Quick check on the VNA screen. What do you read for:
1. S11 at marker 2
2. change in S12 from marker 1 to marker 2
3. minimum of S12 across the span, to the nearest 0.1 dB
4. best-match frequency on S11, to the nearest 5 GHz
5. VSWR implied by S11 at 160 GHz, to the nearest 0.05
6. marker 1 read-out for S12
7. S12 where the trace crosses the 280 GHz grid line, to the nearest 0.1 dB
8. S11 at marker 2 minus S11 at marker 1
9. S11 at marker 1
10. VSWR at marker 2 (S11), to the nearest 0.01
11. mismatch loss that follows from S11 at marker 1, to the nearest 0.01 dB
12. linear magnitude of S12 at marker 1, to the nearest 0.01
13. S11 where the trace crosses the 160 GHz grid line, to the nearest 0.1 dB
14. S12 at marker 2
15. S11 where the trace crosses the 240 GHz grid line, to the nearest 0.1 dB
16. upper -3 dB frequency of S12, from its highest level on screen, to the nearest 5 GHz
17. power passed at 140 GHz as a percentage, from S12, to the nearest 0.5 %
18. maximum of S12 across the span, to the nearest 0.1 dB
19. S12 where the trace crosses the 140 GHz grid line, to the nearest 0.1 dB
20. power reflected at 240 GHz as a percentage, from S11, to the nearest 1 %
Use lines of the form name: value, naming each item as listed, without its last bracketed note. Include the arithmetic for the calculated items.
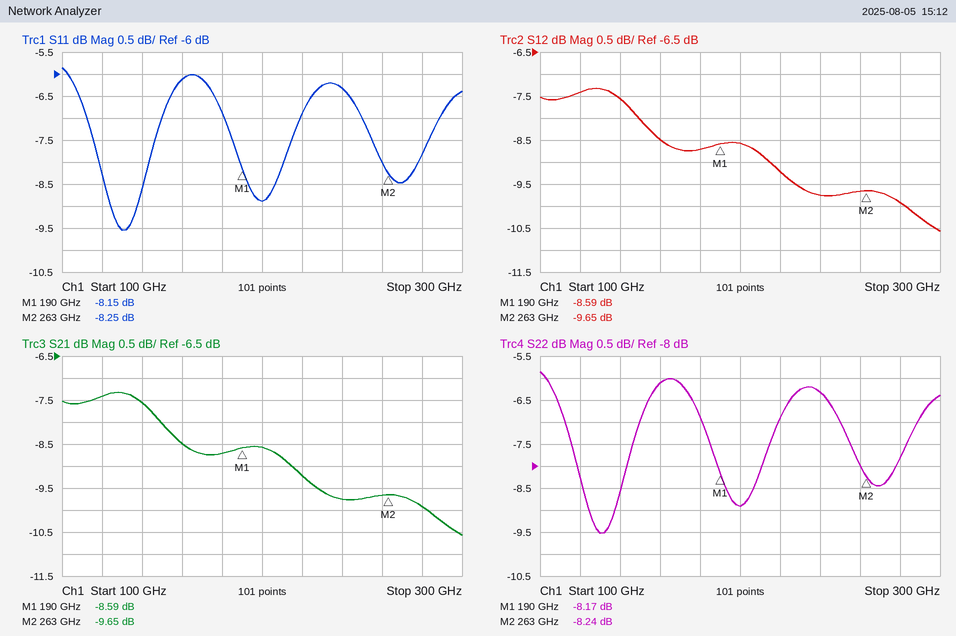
S11 at marker 2: -8.25 dB
change in S12 from marker 1 to marker 2: -9.65 − (-8.59) = -1.06 dB
minimum of S12 across the span, to the nearest 0.1 dB: -10.6 dB
best-match frequency on S11, to the nearest 5 GHz: 130 GHz
VSWR implied by S11 at 160 GHz, to the nearest 0.05: |Γ| = 10^(-6.1/20) = 0.4955; VSWR = (1 + 0.4955)/(1 − 0.4955) ≈ 2.96, so 2.95 to the nearest 0.05
marker 1 read-out for S12: -8.59 dB
S12 where the trace crosses the 280 GHz grid line, to the nearest 0.1 dB: -9.9 dB
S11 at marker 2 minus S11 at marker 1: -8.25 − (-8.15) = -0.10 dB
S11 at marker 1: -8.15 dB
VSWR at marker 2 (S11), to the nearest 0.01: (1 + 0.3868)/(1 − 0.3868) ≈ 2.26
mismatch loss that follows from S11 at marker 1, to the nearest 0.01 dB: −10 log10(1 − 10^(-8.15/10)) ≈ 0.72 dB
linear magnitude of S12 at marker 1, to the nearest 0.01: 10^(-8.59/20) ≈ 0.37
S11 where the trace crosses the 160 GHz grid line, to the nearest 0.1 dB: -6.1 dB
S12 at marker 2: -9.65 dB
S11 where the trace crosses the 240 GHz grid line, to the nearest 0.1 dB: -6.3 dB
upper -3 dB frequency of S12, from its highest level on screen, to the nearest 5 GHz: 290 GHz
power passed at 140 GHz as a percentage, from S12, to the nearest 0.5 %: 10^(-7.6/10) ≈ 17.4 %, so 17.5 % to the nearest 0.5 %
maximum of S12 across the span, to the nearest 0.1 dB: -7.3 dB
S12 where the trace crosses the 140 GHz grid line, to the nearest 0.1 dB: -7.6 dB
power reflected at 240 GHz as a percentage, from S11, to the nearest 1 %: 10^(-6.3/10) ≈ 23 %
